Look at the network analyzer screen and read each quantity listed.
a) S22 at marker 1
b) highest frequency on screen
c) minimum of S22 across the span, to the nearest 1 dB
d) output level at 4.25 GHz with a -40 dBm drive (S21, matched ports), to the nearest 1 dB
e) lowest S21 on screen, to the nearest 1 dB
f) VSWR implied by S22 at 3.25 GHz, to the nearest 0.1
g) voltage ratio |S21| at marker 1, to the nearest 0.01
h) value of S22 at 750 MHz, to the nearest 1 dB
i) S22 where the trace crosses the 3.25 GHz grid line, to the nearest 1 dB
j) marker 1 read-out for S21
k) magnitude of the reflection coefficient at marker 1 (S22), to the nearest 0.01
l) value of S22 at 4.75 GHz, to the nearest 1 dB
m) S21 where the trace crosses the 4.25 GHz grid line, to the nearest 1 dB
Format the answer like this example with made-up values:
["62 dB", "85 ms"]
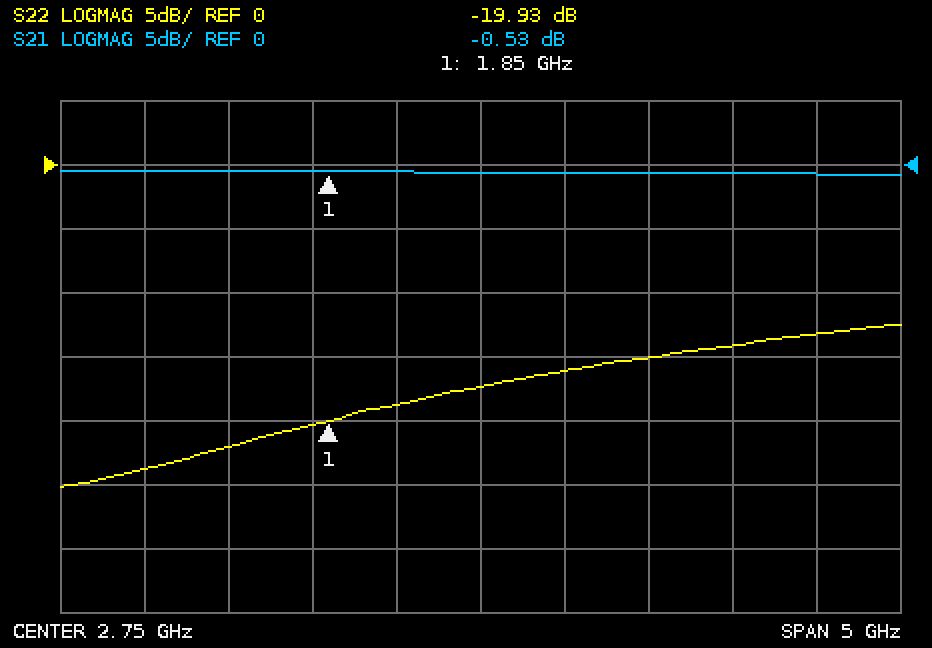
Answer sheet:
["-19.93 dB", "5.25 GHz", "-25 dB", "-41 dBm", "-1 dB", "1.4", "0.94", "-24 dB", "-16 dB", "-0.53 dB", "0.10", "-13 dB", "-1 dB"]
